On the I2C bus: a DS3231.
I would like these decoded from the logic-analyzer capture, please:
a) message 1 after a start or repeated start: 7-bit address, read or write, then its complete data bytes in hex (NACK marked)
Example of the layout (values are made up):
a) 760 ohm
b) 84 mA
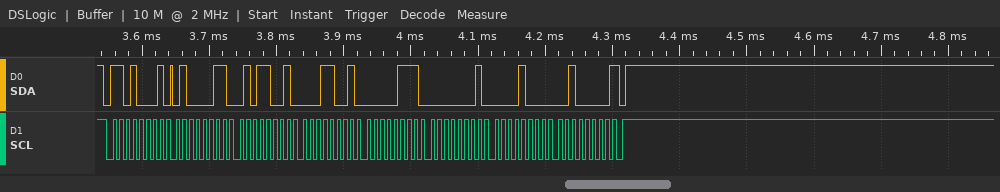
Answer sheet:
a) 0x68 read: 43 59 19 07 01 08 20 NACK
